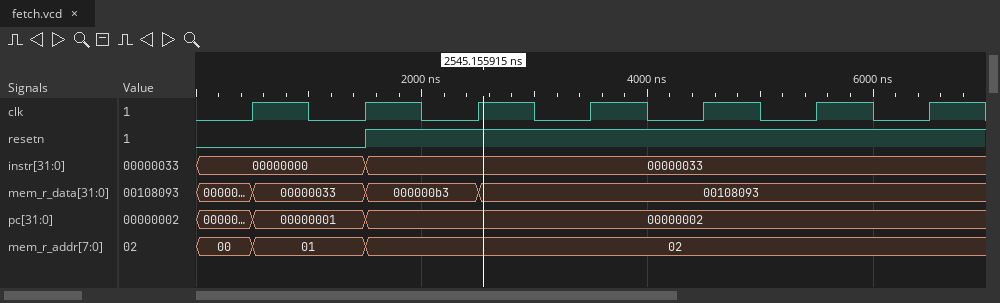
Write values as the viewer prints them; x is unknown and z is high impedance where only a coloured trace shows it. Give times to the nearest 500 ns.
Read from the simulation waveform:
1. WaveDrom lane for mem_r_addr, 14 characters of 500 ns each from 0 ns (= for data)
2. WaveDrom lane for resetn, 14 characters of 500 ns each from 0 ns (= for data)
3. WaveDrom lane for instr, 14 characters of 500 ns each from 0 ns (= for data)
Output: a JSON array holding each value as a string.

["{name: 'mem_r_addr', wave: '==.=..........', data: '00 01 02'}", "{name: 'resetn', wave: '0..1..........'}", "{name: 'instr', wave: '=..=..........', data: '00000000 00000033'}"]
